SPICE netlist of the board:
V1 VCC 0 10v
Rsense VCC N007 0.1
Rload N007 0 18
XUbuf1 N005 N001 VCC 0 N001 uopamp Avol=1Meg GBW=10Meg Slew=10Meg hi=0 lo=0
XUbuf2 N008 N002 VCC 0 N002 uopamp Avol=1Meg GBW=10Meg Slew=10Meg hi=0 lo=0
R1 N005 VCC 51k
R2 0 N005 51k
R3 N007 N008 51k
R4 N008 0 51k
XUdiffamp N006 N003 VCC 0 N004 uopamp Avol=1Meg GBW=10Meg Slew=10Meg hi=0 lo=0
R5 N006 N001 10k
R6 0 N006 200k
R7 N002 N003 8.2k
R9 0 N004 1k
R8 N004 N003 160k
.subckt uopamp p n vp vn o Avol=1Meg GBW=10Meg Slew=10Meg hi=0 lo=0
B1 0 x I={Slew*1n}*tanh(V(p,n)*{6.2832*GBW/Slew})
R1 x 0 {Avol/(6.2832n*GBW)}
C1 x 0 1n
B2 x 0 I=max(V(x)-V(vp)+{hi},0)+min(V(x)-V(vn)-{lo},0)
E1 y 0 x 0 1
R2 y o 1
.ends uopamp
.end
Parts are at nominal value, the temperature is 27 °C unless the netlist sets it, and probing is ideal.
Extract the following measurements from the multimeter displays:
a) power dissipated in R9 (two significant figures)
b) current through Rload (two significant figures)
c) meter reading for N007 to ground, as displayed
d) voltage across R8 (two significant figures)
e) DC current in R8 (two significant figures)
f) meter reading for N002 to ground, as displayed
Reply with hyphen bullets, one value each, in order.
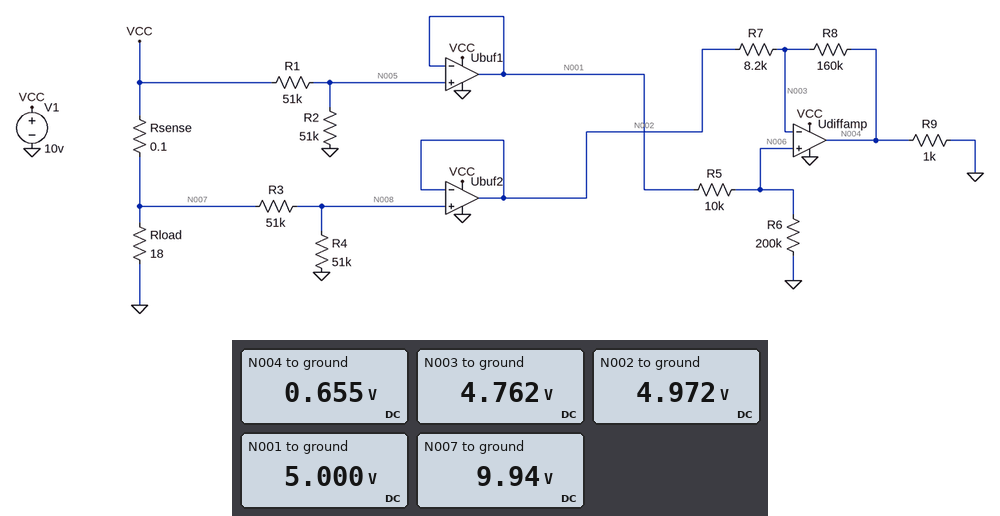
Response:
- 430 µW
- 550 mA
- 9.94 V
- 4.1 V
- 26 µA
- 4.972 V
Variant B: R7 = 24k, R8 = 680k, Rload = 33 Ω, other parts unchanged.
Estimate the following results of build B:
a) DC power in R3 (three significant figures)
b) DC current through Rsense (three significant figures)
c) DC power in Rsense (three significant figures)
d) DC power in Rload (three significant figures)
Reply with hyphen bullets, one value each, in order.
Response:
- 487 µW
- 302 mA
- 9.13 mW
- 3.01 W
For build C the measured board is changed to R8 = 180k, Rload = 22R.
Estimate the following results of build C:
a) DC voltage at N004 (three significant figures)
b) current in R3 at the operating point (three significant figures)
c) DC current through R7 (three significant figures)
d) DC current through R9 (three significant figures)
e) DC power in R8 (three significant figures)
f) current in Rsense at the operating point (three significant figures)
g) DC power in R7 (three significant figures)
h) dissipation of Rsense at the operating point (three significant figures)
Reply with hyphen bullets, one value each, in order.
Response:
- 32.2 mV
- 97.6 µA
- 26.3 µA
- 32.2 µA
- 124 µW
- 453 mA
- 5.66 µW
- 20.5 mW
